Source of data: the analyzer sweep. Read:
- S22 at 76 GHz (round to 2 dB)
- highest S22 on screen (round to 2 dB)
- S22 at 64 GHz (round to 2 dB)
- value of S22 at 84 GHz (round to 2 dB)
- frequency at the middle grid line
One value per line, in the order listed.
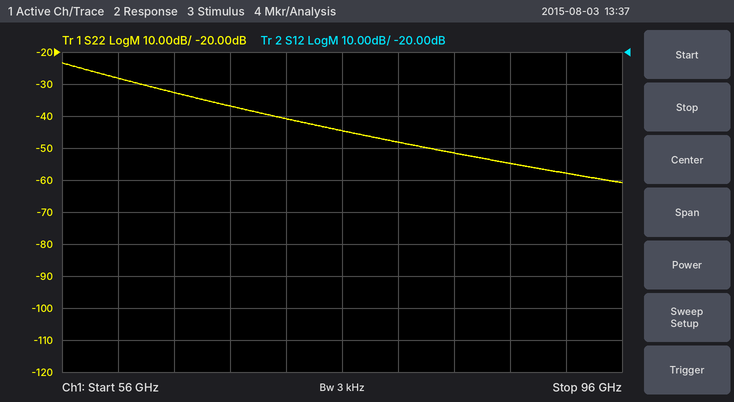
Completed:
-44 dB
-24 dB
-32 dB
-52 dB
76 GHz
